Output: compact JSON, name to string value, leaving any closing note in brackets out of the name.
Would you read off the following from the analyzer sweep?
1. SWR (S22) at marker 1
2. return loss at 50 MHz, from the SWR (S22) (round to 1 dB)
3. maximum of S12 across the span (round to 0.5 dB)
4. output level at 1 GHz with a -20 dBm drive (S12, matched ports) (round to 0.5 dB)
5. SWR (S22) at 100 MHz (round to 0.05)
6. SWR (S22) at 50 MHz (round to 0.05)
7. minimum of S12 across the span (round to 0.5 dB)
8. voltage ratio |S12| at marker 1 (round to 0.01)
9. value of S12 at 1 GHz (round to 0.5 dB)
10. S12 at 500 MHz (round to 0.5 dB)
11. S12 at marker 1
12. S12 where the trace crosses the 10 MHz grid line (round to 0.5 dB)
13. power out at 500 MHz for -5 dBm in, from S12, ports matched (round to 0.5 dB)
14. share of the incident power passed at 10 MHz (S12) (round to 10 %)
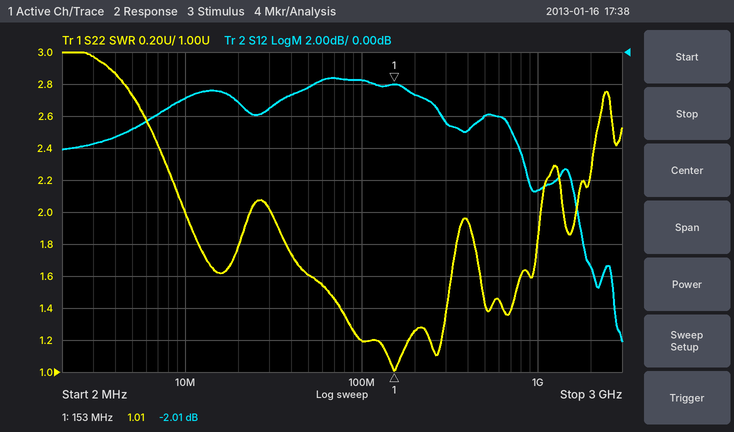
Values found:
{"SWR (S22) at marker 1": "1.01", "return loss at 50 MHz, from the SWR (S22)": "13 dB", "maximum of S12 across the span": "-1.5 dB", "output level at 1 GHz with a -20 dBm drive (S12, matched ports)": "-28.5 dBm", "SWR (S22) at 100 MHz": "1.20", "SWR (S22) at 50 MHz": "1.60", "minimum of S12 across the span": "-18.0 dB", "voltage ratio |S12| at marker 1": "0.79", "value of S12 at 1 GHz": "-8.5 dB", "S12 at 500 MHz": "-4.0 dB", "S12 at marker 1": "-2.01 dB", "S12 where the trace crosses the 10 MHz grid line": "-3.0 dB", "power out at 500 MHz for -5 dBm in, from S12, ports matched": "-9.0 dBm", "share of the incident power passed at 10 MHz (S12)": "50 %"}
